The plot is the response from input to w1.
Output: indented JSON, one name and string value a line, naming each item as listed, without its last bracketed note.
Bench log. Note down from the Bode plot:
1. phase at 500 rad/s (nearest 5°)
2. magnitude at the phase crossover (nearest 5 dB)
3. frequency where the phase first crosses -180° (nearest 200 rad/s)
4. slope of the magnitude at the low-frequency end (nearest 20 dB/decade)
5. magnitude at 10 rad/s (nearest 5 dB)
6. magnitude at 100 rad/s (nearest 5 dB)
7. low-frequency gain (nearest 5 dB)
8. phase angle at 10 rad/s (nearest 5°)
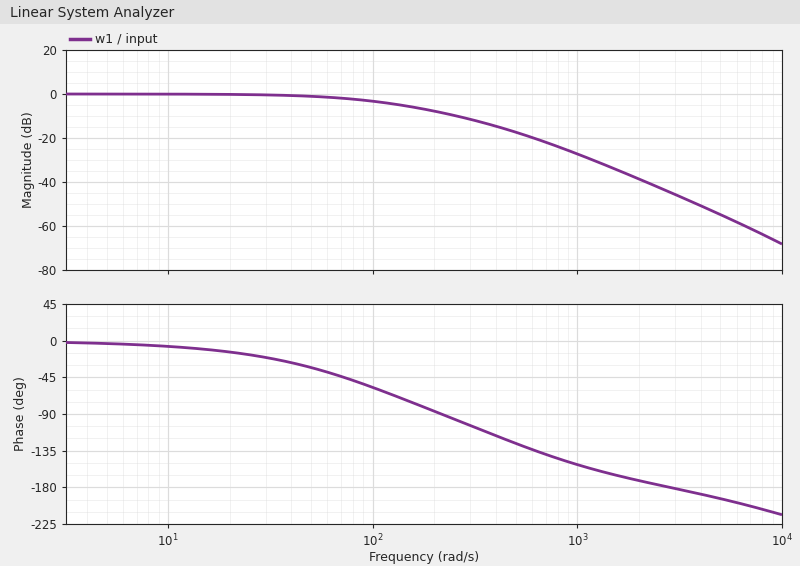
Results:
{
  "phase at 500 rad/s": "-125°",
  "magnitude at the phase crossover": "-45 dB",
  "frequency where the phase first crosses -180°": "2800 rad/s",
  "slope of the magnitude at the low-frequency end": "0 dB/decade",
  "magnitude at 10 rad/s": "0 dB",
  "magnitude at 100 rad/s": "-5 dB",
  "low-frequency gain": "0 dB",
  "phase angle at 10 rad/s": "-5°"
}
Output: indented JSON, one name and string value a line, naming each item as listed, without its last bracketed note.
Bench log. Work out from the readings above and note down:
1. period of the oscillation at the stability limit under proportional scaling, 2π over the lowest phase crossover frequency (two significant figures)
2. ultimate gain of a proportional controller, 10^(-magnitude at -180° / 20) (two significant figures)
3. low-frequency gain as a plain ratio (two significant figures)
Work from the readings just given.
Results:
{
  "period of the oscillation at the stability limit under proportional scaling, 2π over the lowest phase crossover frequency": "0.0022 s",
  "ultimate gain of a proportional controller, 10^(-magnitude at -180° / 20)": "180",
  "low-frequency gain as a plain ratio": "1.0"
}
